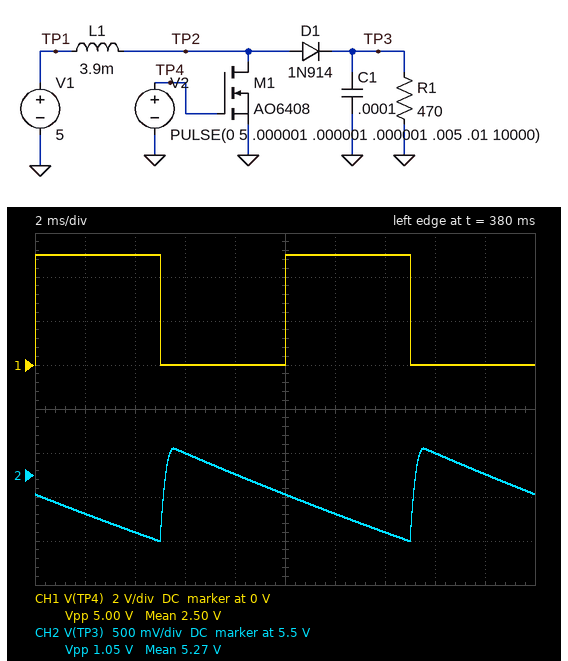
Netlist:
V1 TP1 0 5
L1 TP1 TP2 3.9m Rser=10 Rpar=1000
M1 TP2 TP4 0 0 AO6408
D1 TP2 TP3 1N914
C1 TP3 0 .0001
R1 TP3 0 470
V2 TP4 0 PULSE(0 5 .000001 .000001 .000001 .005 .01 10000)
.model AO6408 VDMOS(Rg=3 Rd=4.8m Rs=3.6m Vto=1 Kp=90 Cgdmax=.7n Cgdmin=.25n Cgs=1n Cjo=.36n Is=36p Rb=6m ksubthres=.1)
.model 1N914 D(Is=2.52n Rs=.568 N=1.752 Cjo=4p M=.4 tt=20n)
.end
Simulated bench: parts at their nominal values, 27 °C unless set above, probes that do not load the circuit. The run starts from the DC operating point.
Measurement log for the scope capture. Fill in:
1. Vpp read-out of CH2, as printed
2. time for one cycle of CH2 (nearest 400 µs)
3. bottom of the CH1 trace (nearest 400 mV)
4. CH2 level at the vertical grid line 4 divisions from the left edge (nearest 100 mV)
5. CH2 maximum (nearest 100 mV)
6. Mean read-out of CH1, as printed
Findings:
1.05 V
10.0 ms
0 V
5.5 V
5.8 V
2.50 V
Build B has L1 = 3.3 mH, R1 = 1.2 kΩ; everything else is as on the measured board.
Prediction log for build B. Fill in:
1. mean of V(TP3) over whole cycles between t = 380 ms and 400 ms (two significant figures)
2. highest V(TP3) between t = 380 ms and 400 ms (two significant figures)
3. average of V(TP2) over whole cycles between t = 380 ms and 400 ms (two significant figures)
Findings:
7.4 V
7.7 V
2.6 V
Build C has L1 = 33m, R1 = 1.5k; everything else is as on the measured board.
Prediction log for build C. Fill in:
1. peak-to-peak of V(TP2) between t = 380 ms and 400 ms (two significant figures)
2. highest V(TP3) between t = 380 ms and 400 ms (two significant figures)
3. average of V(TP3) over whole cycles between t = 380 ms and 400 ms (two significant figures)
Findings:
21 V
20 V
19 V
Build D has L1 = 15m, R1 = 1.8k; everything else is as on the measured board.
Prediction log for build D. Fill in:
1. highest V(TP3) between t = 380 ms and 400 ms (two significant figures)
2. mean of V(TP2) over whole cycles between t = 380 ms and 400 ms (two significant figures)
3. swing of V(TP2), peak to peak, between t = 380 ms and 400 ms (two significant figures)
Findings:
18 V
3.1 V
19 V
